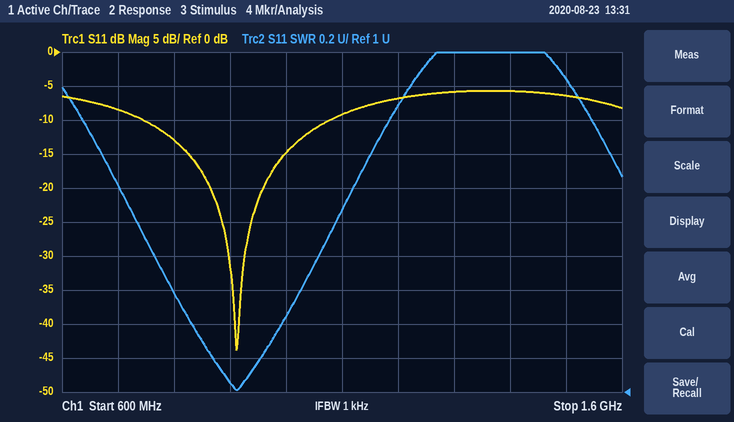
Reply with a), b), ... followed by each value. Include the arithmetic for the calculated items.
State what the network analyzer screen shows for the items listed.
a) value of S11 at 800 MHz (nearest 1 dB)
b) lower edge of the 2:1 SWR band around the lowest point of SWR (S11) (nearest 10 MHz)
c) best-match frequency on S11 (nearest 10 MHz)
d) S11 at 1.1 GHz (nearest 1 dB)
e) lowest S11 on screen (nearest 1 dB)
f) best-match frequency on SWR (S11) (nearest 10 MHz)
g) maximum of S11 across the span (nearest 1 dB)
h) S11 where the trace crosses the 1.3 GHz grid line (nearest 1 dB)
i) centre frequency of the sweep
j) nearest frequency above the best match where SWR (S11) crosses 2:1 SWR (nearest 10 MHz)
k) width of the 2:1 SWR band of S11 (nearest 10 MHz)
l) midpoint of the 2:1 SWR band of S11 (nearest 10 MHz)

a) -13 dB
b) 730 MHz
c) 910 MHz
d) -9 dB
e) -44 dB
f) 910 MHz
g) -6 dB
h) -6 dB
i) 1.1 GHz
j) 1.09 GHz
k) 1.09 GHz − 730 MHz = 360 MHz
l) 910 MHz
